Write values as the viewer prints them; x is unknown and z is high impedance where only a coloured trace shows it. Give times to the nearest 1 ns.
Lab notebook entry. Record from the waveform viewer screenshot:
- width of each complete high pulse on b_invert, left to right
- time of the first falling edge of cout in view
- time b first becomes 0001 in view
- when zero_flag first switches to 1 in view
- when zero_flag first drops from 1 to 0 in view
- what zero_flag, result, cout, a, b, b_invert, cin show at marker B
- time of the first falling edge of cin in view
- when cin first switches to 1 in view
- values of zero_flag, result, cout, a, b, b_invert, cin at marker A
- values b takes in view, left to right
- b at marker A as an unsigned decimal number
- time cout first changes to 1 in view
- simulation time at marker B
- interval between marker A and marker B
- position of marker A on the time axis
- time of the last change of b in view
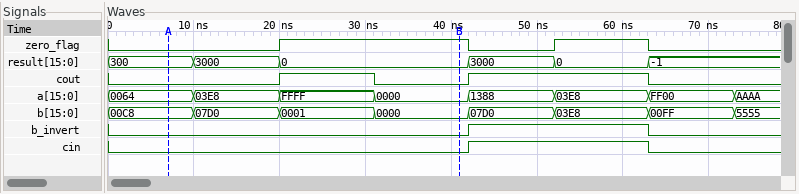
21 ns
31 ns
20 ns
20 ns
42 ns
zero_flag=1, result=0, cout=0, a=0000, b=0000, b_invert=0, cin=0
63 ns
42 ns
zero_flag=0, result=300, cout=0, a=0064, b=00C8, b_invert=0, cin=0
00C8, 07D0, 0001, 0000, 07D0, 03E8, 00FF, 5555
200
20 ns
41 ns
34 ns
7 ns
73 ns
